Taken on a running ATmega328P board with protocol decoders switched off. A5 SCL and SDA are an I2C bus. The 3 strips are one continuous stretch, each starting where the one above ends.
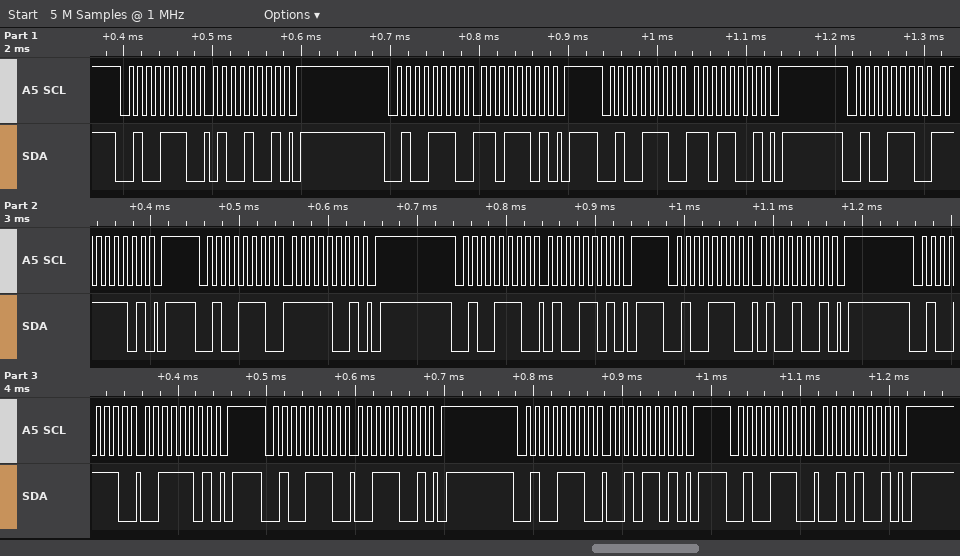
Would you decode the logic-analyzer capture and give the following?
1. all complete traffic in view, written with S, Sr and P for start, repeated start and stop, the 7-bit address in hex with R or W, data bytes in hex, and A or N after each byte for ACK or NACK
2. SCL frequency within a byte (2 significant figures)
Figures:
S 27W A 49 A P S 27W A DD A P S 27W A D9 A P S 27W A FD A P S 27W A F9 A P S 27W A 4D A P S 27W A 49 A P S 27W A 3D A P S 27W A 39 A P S 27W A 2D A P S 27W A 29 A P
100 kHz
